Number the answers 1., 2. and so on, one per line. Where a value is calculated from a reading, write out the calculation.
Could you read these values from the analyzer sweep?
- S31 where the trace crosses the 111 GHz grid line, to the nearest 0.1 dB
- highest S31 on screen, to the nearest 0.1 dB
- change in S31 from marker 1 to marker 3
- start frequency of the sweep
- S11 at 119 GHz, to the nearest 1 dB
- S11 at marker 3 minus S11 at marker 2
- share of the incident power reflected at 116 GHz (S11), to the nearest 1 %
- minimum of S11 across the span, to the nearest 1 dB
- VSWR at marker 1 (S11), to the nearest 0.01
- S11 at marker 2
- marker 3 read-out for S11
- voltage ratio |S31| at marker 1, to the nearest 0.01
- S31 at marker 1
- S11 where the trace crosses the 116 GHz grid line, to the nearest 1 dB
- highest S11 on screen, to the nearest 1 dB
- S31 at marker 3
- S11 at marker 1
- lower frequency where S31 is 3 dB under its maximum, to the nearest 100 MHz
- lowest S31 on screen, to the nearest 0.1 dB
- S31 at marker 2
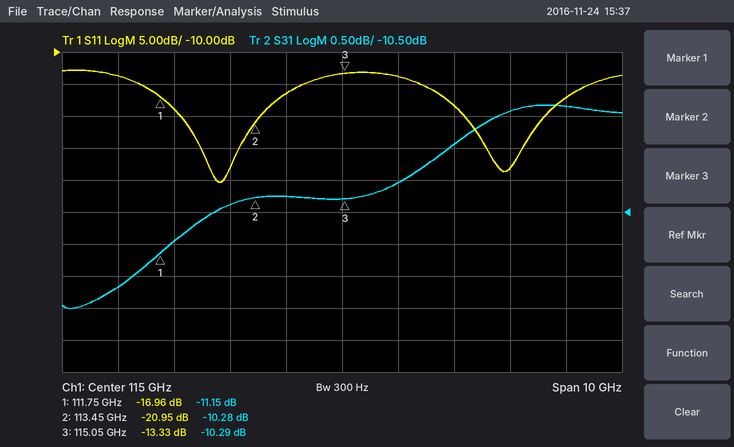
1. -11.7 dB
2. -8.8 dB
3. -10.29 − (-11.15) = 0.86 dB
4. 110 GHz
5. -17 dB
6. -13.33 − (-20.95) = 7.62 dB
7. 10^(-14/10) ≈ 4 %
8. -30 dB
9. (1 + 0.1419)/(1 − 0.1419) ≈ 1.33
10. -20.95 dB
11. -13.33 dB
12. 10^(-11.15/20) ≈ 0.28
13. -11.15 dB
14. -14 dB
15. -13 dB
16. -10.29 dB
17. -16.96 dB
18. 110.7 GHz
19. -12.0 dB
20. -10.28 dB
